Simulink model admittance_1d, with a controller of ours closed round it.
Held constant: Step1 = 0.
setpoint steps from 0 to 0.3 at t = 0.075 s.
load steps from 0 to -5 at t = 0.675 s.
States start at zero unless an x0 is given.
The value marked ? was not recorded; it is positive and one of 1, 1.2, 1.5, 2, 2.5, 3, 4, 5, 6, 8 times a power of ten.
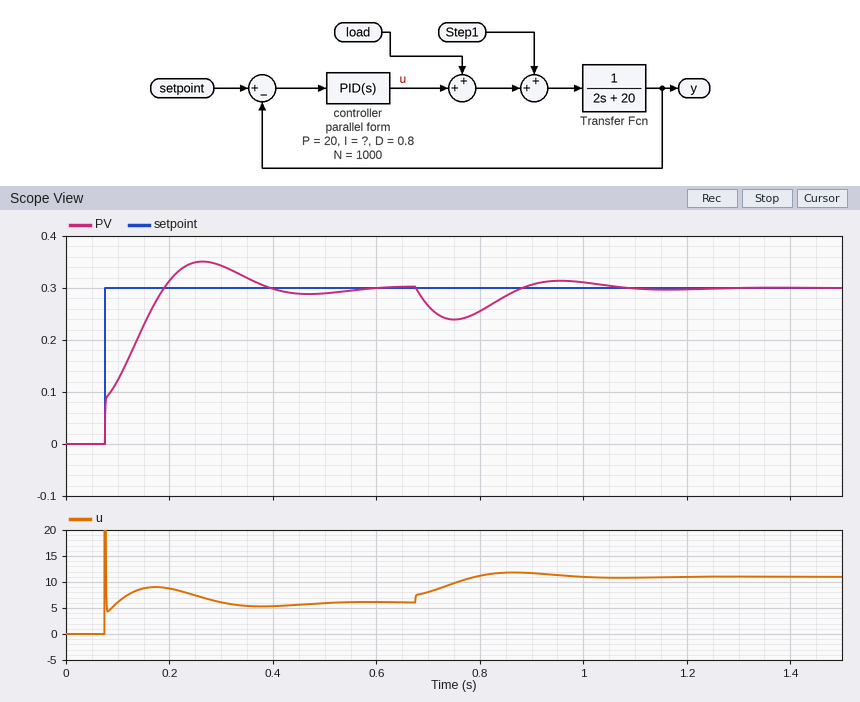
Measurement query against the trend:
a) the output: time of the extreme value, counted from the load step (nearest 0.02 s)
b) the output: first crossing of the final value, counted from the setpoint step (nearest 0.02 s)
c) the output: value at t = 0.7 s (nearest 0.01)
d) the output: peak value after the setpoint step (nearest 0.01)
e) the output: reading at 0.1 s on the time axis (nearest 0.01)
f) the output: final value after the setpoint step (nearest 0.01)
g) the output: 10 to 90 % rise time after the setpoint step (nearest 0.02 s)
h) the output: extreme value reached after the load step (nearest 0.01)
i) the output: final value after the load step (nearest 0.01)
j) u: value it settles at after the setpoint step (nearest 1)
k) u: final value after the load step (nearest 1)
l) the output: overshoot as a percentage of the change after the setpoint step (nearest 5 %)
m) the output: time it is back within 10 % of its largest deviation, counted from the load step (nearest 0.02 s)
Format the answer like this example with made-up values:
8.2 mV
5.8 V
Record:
0.08 s
0.12 s
0.27
0.35
0.12
0.30
0.10 s
0.24
0.30
6
11
15 %
0.36 s
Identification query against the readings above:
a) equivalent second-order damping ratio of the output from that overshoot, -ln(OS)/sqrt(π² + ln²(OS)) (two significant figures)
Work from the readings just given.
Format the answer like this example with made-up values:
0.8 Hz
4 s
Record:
0.52
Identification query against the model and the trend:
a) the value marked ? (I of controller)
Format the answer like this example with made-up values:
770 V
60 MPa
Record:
800
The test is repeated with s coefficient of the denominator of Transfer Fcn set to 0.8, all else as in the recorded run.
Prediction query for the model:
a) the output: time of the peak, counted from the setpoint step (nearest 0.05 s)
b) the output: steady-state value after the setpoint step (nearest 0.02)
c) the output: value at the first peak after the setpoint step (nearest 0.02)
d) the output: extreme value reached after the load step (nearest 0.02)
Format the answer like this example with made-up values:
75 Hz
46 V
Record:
0.15 s
0.30
0.32
0.22
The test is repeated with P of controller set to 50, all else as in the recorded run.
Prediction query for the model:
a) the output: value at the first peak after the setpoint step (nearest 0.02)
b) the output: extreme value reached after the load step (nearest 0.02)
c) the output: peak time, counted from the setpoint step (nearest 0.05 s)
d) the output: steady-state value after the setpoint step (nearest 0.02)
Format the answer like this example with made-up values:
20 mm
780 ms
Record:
0.32
0.26
0.20 s
0.30
